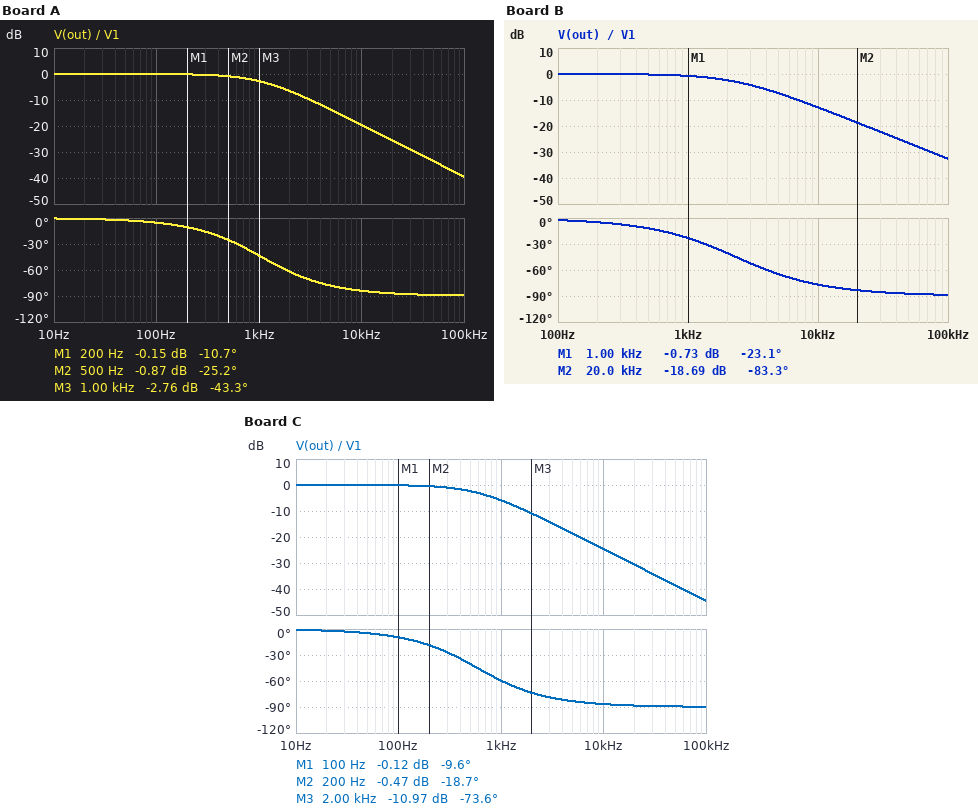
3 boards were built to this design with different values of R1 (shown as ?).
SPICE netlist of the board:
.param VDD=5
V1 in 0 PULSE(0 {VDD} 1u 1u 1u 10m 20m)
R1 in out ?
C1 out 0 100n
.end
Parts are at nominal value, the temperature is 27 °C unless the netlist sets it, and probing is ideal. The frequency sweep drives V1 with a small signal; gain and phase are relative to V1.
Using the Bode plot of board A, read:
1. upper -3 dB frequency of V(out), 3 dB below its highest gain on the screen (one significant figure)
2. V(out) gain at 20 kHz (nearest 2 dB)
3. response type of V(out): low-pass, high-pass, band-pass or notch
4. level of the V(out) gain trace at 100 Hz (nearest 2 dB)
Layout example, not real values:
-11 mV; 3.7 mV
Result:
1 kHz; -26 dB; low-pass; 0 dB
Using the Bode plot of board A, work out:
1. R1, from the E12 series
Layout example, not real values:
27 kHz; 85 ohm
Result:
1.5 kΩ
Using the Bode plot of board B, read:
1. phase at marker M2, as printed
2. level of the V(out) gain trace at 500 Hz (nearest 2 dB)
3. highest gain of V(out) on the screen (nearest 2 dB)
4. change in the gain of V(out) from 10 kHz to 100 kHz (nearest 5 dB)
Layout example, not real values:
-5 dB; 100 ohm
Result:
-83.3 deg; 0 dB; 0 dB; -20 dB
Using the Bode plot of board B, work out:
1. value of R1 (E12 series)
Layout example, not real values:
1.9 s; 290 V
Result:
680 Ω
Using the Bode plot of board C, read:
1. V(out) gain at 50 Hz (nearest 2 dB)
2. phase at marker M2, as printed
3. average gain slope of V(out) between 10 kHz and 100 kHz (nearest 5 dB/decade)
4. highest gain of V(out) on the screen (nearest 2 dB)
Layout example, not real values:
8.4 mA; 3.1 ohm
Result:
0 dB; -18.7 deg; -20 dB/decade; 0 dB
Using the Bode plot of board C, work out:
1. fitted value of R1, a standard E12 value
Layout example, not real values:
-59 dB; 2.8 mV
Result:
2.7 kΩ
